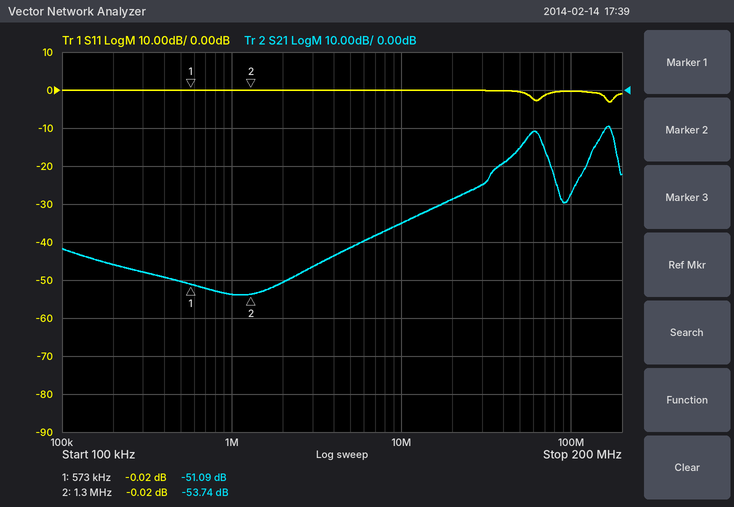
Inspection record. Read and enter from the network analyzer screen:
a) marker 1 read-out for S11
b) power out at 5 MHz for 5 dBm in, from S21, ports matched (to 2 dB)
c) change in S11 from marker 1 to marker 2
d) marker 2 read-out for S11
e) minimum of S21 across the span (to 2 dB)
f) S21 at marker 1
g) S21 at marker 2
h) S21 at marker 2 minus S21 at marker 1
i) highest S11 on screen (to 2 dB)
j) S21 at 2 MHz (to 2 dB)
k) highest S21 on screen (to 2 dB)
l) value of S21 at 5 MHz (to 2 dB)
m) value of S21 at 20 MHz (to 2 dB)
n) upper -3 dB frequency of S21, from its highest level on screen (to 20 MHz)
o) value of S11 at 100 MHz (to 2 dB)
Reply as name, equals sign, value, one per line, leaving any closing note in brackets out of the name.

marker 1 read-out for S11 = -0.02 dB
power out at 5 MHz for 5 dBm in, from S21, ports matched = -36 dBm
change in S11 from marker 1 to marker 2 = 0.00 dB
marker 2 read-out for S11 = -0.02 dB
minimum of S21 across the span = -54 dB
S21 at marker 1 = -51.09 dB
S21 at marker 2 = -53.74 dB
S21 at marker 2 minus S21 at marker 1 = -2.65 dB
highest S11 on screen = 0 dB
S21 at 2 MHz = -50 dB
highest S21 on screen = -10 dB
value of S21 at 5 MHz = -42 dB
value of S21 at 20 MHz = -28 dB
upper -3 dB frequency of S21, from its highest level on screen = 180 MHz
value of S11 at 100 MHz = 0 dB
